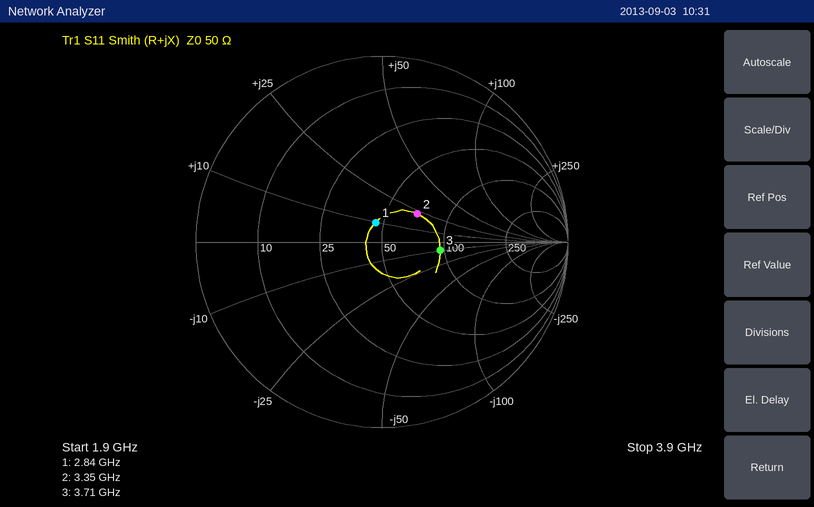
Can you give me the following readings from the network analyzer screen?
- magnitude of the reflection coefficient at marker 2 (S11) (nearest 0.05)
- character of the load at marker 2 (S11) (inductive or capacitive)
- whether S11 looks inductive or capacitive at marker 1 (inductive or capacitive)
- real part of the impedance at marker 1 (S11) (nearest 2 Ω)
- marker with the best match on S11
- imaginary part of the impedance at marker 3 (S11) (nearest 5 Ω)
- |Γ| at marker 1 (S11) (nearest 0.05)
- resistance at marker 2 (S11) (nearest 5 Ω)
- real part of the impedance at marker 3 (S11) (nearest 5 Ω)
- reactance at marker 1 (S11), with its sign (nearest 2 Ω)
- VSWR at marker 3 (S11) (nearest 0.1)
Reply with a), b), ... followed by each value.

a) 0.25
b) inductive
c) inductive
d) 46 Ω
e) marker 1
f) -10 Ω
g) 0.10
h) 70 Ω
i) 95 Ω
j) +10 Ω
k) 1.9
